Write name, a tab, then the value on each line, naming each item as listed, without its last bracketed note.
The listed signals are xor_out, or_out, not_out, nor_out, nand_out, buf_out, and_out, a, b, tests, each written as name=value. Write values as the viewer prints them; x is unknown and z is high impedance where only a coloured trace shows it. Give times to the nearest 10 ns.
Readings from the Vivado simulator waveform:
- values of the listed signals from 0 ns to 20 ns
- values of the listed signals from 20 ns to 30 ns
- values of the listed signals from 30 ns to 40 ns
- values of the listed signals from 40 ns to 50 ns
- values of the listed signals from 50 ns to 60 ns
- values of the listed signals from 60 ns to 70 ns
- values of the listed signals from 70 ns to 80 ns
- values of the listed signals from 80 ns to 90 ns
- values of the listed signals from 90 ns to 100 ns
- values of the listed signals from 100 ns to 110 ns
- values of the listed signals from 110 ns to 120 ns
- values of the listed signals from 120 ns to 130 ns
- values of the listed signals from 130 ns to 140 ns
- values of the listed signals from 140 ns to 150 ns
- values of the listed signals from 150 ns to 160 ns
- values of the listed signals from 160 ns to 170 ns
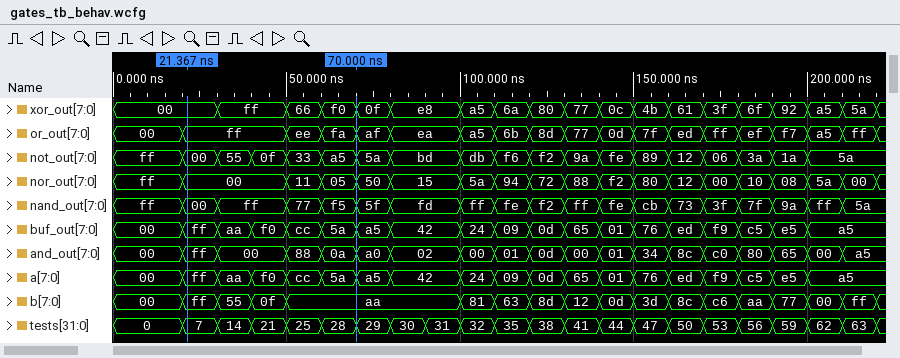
values of the listed signals from 0 ns to 20 ns	xor_out=00, or_out=00, not_out=ff, nor_out=ff, nand_out=ff, buf_out=00, and_out=00, a=00, b=00, tests=0
values of the listed signals from 20 ns to 30 ns	xor_out=00, or_out=ff, not_out=00, nor_out=00, nand_out=00, buf_out=ff, and_out=ff, a=ff, b=ff, tests=7
values of the listed signals from 30 ns to 40 ns	xor_out=ff, or_out=ff, not_out=55, nor_out=00, nand_out=ff, buf_out=aa, and_out=00, a=aa, b=55, tests=14
values of the listed signals from 40 ns to 50 ns	xor_out=ff, or_out=ff, not_out=0f, nor_out=00, nand_out=ff, buf_out=f0, and_out=00, a=f0, b=0f, tests=21
values of the listed signals from 50 ns to 60 ns	xor_out=66, or_out=ee, not_out=33, nor_out=11, nand_out=77, buf_out=cc, and_out=88, a=cc, b=aa, tests=25
values of the listed signals from 60 ns to 70 ns	xor_out=f0, or_out=fa, not_out=a5, nor_out=05, nand_out=f5, buf_out=5a, and_out=0a, a=5a, b=aa, tests=28
values of the listed signals from 70 ns to 80 ns	xor_out=0f, or_out=af, not_out=5a, nor_out=50, nand_out=5f, buf_out=a5, and_out=a0, a=a5, b=aa, tests=29
values of the listed signals from 80 ns to 90 ns	xor_out=e8, or_out=ea, not_out=bd, nor_out=15, nand_out=fd, buf_out=42, and_out=02, a=42, b=aa, tests=30
values of the listed signals from 90 ns to 100 ns	xor_out=e8, or_out=ea, not_out=bd, nor_out=15, nand_out=fd, buf_out=42, and_out=02, a=42, b=aa, tests=31
values of the listed signals from 100 ns to 110 ns	xor_out=a5, or_out=a5, not_out=db, nor_out=5a, nand_out=ff, buf_out=24, and_out=00, a=24, b=81, tests=32
values of the listed signals from 110 ns to 120 ns	xor_out=6a, or_out=6b, not_out=f6, nor_out=94, nand_out=fe, buf_out=09, and_out=01, a=09, b=63, tests=35
values of the listed signals from 120 ns to 130 ns	xor_out=80, or_out=8d, not_out=f2, nor_out=72, nand_out=f2, buf_out=0d, and_out=0d, a=0d, b=8d, tests=38
values of the listed signals from 130 ns to 140 ns	xor_out=77, or_out=77, not_out=9a, nor_out=88, nand_out=ff, buf_out=65, and_out=00, a=65, b=12, tests=41
values of the listed signals from 140 ns to 150 ns	xor_out=0c, or_out=0d, not_out=fe, nor_out=f2, nand_out=fe, buf_out=01, and_out=01, a=01, b=0d, tests=44
values of the listed signals from 150 ns to 160 ns	xor_out=4b, or_out=7f, not_out=89, nor_out=80, nand_out=cb, buf_out=76, and_out=34, a=76, b=3d, tests=47
values of the listed signals from 160 ns to 170 ns	xor_out=61, or_out=ed, not_out=12, nor_out=12, nand_out=73, buf_out=ed, and_out=8c, a=ed, b=8c, tests=50
